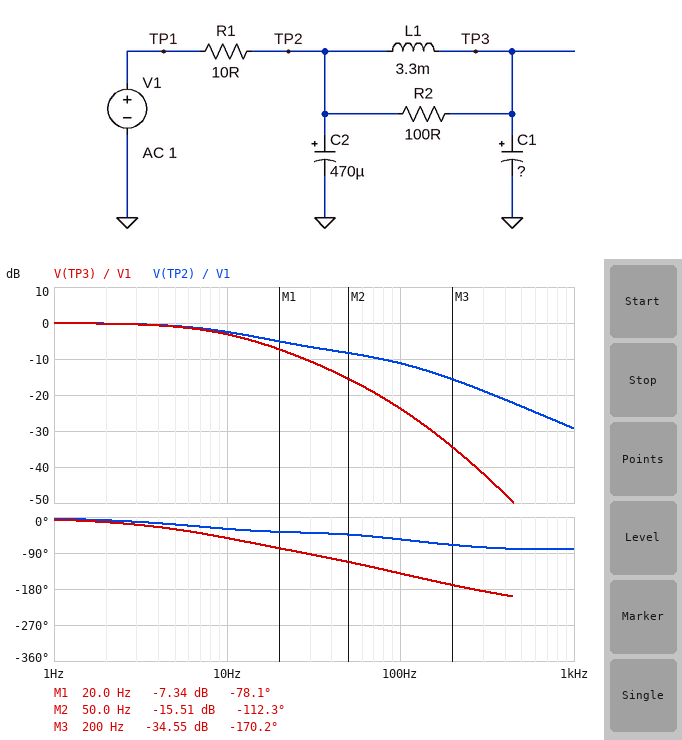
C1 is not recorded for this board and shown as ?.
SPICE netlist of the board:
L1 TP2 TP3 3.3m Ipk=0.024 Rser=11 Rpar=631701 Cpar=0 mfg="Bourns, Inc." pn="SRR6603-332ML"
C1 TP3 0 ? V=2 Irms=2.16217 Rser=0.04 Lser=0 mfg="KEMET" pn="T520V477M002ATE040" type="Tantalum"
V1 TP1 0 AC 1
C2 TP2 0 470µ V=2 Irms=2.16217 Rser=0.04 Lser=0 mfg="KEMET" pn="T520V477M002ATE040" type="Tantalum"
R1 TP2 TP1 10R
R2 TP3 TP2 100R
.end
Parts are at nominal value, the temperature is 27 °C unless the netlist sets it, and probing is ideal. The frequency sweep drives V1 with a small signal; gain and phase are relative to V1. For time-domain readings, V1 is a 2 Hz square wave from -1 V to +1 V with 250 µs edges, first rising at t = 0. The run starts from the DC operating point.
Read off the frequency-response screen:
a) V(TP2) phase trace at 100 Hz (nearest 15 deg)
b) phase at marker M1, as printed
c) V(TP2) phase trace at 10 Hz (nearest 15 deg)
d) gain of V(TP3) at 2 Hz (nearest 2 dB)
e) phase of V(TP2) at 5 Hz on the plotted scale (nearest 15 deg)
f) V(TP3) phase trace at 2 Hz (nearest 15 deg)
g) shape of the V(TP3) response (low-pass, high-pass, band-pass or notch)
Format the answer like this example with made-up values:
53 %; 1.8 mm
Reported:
-60 deg; -78.1 deg; -30 deg; 0 dB; -15 deg; -15 deg; low-pass
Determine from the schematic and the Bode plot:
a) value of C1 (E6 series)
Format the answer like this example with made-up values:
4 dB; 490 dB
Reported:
680 µF
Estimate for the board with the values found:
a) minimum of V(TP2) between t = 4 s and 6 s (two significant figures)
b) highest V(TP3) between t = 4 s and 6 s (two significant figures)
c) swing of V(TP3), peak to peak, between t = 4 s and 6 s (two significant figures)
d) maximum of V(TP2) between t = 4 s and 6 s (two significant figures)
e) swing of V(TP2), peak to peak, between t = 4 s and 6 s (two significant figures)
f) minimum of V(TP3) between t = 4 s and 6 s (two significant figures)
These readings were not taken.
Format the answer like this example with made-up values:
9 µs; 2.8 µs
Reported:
-1.0 V; 1.0 V; 2.0 V; 1.0 V; 2.0 V; -1.0 V
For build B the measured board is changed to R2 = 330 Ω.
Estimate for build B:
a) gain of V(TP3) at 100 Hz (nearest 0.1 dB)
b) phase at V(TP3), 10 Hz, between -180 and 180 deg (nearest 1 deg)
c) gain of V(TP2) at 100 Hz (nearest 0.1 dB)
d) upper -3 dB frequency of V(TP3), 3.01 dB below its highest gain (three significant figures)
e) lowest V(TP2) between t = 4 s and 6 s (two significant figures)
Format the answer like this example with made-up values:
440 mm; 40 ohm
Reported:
-24.3 dB; -54 deg; -11.1 dB; 9.46 Hz; -1.0 V
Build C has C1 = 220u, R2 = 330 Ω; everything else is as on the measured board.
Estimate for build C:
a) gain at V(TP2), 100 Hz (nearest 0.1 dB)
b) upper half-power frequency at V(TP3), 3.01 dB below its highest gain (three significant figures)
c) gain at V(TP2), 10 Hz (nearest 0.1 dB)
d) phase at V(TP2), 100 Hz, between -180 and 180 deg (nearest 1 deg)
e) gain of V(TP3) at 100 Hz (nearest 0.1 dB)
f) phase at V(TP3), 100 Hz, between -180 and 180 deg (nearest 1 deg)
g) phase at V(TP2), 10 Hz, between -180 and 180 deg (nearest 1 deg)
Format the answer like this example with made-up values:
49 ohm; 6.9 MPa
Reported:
-11.5 dB; 20.0 Hz; -0.9 dB; -62 deg; -15.9 dB; -125 deg; -23 deg
